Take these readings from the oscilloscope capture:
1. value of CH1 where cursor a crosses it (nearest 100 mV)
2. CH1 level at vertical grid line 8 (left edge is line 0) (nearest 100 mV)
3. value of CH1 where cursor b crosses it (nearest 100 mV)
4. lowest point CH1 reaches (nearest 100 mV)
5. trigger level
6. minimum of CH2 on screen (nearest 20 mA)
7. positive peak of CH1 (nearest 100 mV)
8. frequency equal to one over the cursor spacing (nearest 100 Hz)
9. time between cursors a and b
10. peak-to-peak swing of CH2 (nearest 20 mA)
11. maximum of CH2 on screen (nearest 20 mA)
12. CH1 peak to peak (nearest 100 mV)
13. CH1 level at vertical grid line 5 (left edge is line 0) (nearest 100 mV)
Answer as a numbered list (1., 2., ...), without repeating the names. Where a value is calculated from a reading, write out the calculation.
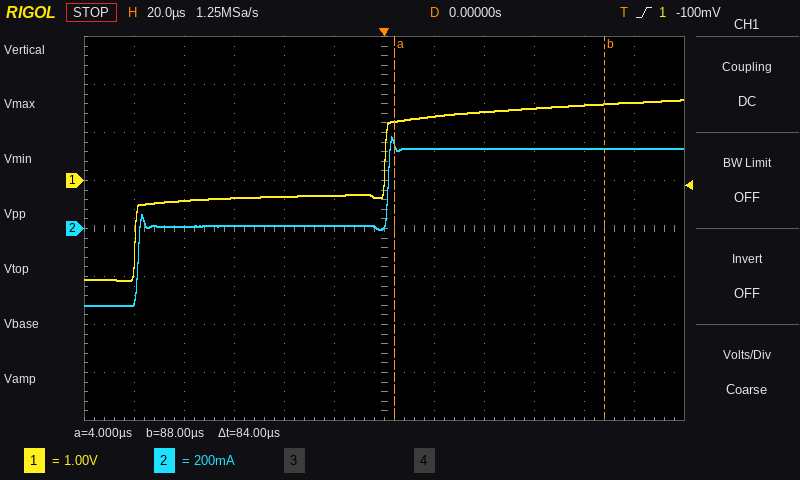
1. 1.2 V
2. 1.4 V
3. 1.6 V
4. -2.1 V
5. -100 mV
6. -320 mA
7. 1.7 V
8. 1 / 84 µs ≈ 11.9 kHz
9. 84 µs
10. 380 mA − (-320 mA) = 700 mA
11. 380 mA
12. 1.7 V − (-2.1 V) = 3.8 V
13. -300 mV
